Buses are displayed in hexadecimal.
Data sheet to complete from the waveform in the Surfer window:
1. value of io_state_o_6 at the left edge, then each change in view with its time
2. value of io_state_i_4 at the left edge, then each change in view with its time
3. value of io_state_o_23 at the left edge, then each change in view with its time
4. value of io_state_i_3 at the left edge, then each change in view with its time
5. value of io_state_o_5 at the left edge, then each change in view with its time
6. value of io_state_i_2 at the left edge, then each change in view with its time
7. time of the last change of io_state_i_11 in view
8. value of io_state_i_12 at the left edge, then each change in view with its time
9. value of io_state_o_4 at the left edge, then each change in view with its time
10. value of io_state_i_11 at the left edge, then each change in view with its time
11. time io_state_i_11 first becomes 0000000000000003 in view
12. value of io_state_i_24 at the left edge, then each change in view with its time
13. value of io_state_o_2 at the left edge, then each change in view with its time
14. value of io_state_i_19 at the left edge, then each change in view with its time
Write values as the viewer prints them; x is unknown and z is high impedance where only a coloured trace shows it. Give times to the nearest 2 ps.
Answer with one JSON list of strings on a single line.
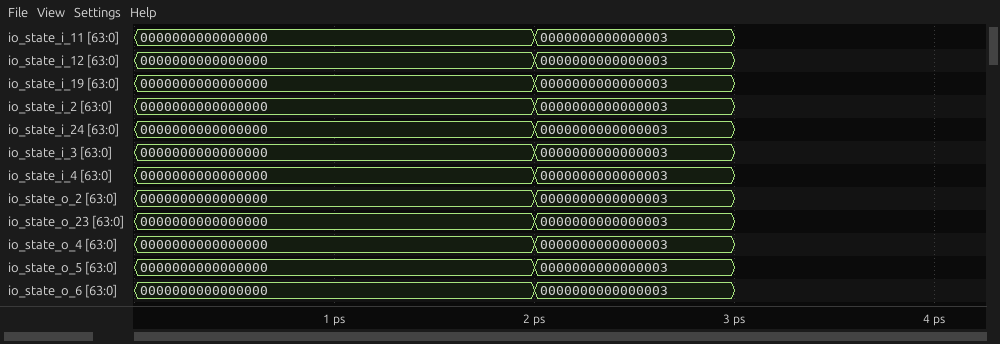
["0000000000000000, 0000000000000003 at 2 ps", "0000000000000000, 0000000000000003 at 2 ps", "0000000000000000, 0000000000000003 at 2 ps", "0000000000000000, 0000000000000003 at 2 ps", "0000000000000000, 0000000000000003 at 2 ps", "0000000000000000, 0000000000000003 at 2 ps", "2 ps", "0000000000000000, 0000000000000003 at 2 ps", "0000000000000000, 0000000000000003 at 2 ps", "0000000000000000, 0000000000000003 at 2 ps", "2 ps", "0000000000000000, 0000000000000003 at 2 ps", "0000000000000000, 0000000000000003 at 2 ps", "0000000000000000, 0000000000000003 at 2 ps"]
